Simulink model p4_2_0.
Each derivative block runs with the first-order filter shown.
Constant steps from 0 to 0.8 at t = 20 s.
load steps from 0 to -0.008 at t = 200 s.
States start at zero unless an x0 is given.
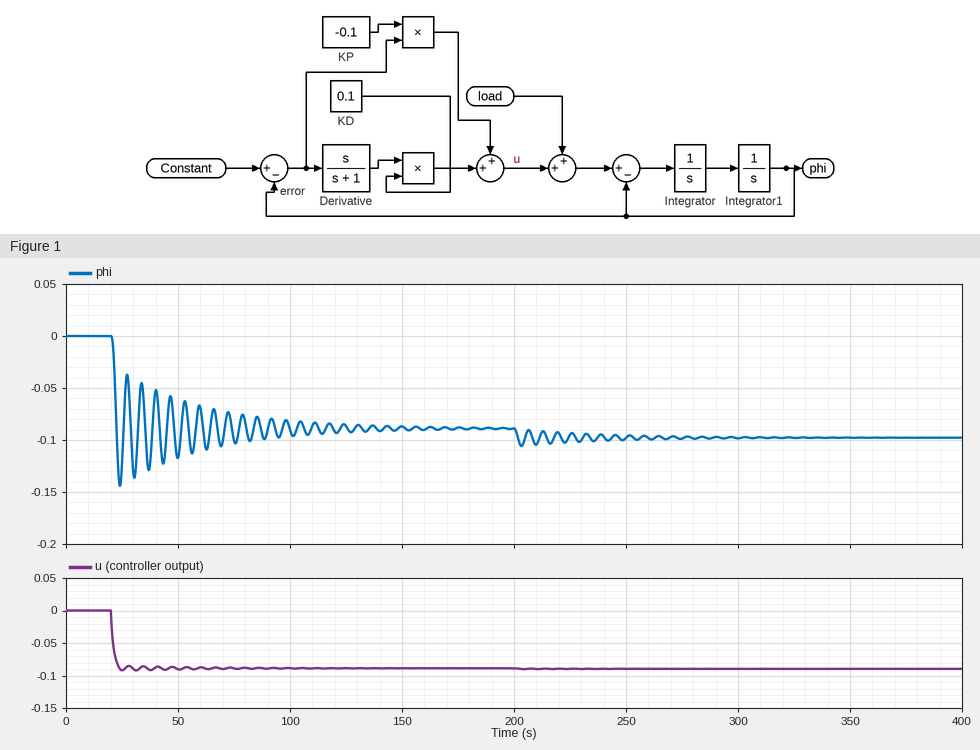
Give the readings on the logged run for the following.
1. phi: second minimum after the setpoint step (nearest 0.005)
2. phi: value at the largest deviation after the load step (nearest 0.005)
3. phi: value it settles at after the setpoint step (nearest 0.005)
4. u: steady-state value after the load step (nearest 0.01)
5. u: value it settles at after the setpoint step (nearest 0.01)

-0.135
-0.105
-0.090
-0.09
-0.09
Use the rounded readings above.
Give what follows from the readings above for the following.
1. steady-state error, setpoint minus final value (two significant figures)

0.89
